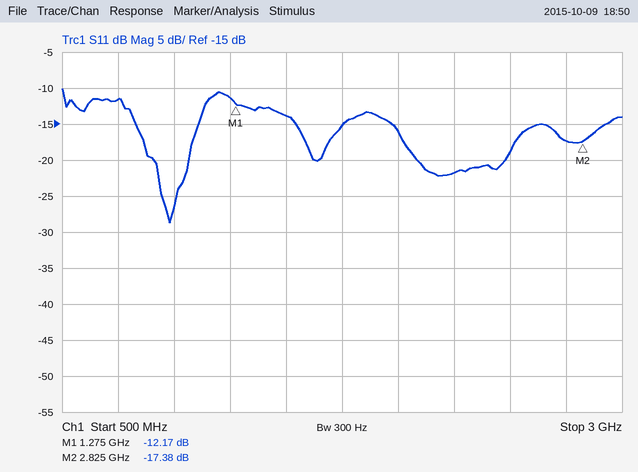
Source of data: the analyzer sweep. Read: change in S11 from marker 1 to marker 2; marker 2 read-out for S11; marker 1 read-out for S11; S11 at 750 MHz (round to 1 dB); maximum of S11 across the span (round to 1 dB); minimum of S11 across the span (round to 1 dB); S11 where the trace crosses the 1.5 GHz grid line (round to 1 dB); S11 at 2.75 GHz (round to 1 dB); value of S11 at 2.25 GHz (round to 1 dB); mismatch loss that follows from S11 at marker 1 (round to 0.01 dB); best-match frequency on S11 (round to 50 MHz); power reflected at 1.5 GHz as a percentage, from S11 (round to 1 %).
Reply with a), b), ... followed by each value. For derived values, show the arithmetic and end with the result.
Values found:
a) -17.38 − (-12.17) = -5.21 dB
b) -17.38 dB
c) -12.17 dB
d) -12 dB
e) -10 dB
f) -29 dB
g) -14 dB
h) -17 dB
i) -22 dB
j) −10 log10(1 − 10^(-12.17/10)) ≈ 0.27 dB
k) 1.00 GHz
l) 10^(-14/10) ≈ 4 %
